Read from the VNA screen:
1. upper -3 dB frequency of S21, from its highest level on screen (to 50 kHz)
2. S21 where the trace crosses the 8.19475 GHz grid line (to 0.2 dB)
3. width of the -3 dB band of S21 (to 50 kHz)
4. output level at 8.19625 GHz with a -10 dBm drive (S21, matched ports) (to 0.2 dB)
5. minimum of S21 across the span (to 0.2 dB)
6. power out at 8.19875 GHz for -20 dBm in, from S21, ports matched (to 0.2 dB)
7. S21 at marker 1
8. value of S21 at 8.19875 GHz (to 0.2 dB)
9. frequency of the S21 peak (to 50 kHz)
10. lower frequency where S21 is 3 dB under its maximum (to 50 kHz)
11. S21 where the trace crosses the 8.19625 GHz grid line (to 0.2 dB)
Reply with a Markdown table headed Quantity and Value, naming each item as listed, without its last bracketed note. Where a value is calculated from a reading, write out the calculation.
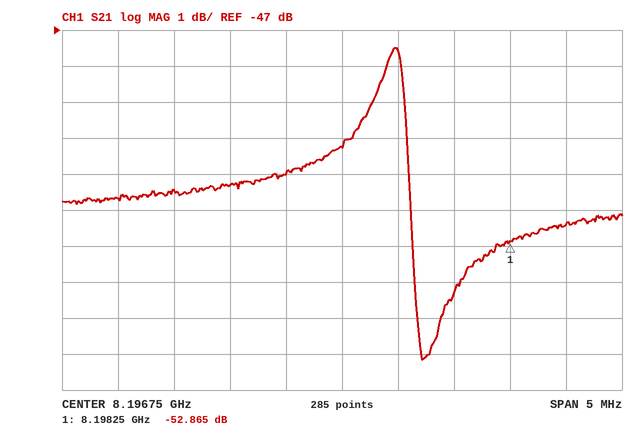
| Quantity | Value |
|---|---|
| upper -3 dB frequency of S21, from its highest level on screen | 8.19735 GHz |
| S21 where the trace crosses the 8.19475 GHz grid line | -51.6 dB |
| width of the -3 dB band of S21 | 8.19735 GHz − 8.19660 GHz = 750 kHz |
| output level at 8.19625 GHz with a -10 dBm drive (S21, matched ports) | -10 dBm + (-51.0 dB) = -61.0 dBm |
| minimum of S21 across the span | -56.2 dB |
| power out at 8.19875 GHz for -20 dBm in, from S21, ports matched | -20 dBm + (-52.4 dB) = -72.4 dBm |
| S21 at marker 1 | -52.865 dB |
| value of S21 at 8.19875 GHz | -52.4 dB |
| frequency of the S21 peak | 8.19720 GHz |
| lower frequency where S21 is 3 dB under its maximum | 8.19660 GHz |
| S21 where the trace crosses the 8.19625 GHz grid line | -51.0 dB |
